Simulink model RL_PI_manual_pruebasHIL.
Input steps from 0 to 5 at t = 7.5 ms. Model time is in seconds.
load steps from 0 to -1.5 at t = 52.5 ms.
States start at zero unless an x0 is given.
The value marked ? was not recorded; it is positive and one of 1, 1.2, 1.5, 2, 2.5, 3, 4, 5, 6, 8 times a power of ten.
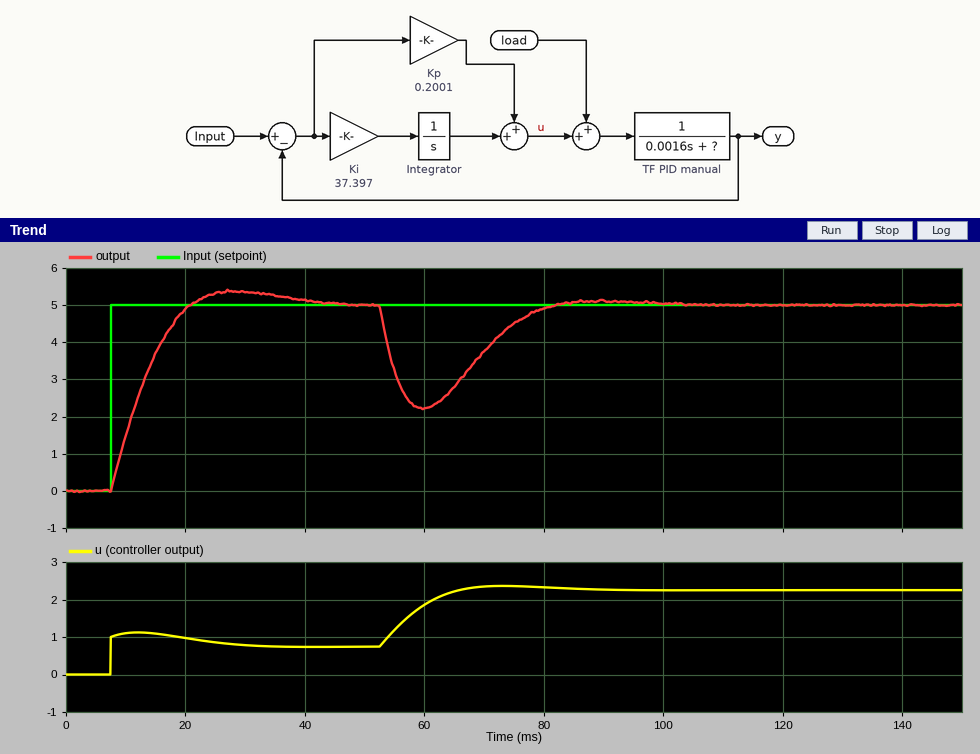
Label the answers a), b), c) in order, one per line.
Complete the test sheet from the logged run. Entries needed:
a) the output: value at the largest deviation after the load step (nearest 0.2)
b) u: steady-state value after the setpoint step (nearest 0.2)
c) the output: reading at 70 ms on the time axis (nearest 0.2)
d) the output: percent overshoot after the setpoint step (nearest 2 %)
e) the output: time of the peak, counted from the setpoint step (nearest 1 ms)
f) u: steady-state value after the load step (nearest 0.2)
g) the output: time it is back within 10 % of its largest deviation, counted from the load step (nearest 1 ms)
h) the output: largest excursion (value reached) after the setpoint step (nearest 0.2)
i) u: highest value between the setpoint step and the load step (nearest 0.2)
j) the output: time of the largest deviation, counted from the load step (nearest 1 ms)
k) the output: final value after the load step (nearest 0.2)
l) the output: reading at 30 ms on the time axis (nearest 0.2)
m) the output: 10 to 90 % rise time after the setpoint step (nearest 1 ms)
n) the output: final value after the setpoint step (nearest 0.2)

a) 2.2
b) 0.8
c) 3.8
d) 8 %
e) 21 ms
f) 2.2
g) 25 ms
h) 5.4
i) 1.2
j) 7 ms
k) 5.0
l) 5.4
m) 10 ms
n) 5.0
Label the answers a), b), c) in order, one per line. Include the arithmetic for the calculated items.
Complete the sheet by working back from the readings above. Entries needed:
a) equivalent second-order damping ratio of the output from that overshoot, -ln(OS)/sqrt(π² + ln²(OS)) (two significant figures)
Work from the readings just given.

a) ln(0.08) = -2.526; 2.526 / sqrt(9.870 + 6.379) = 0.63
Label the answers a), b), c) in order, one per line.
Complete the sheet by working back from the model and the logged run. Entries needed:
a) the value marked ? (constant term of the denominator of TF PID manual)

a) 0.15
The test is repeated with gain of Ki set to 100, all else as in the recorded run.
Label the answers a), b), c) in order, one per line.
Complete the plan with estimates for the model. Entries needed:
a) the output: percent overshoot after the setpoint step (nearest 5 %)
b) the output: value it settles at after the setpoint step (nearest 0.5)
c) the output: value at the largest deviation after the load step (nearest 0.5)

a) 25 %
b) 5.0
c) 3.0
